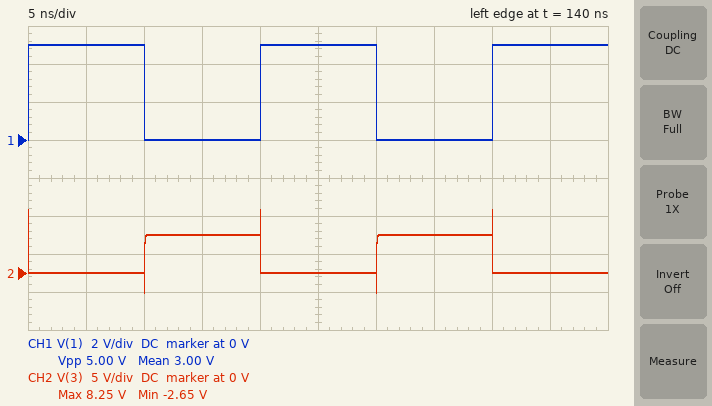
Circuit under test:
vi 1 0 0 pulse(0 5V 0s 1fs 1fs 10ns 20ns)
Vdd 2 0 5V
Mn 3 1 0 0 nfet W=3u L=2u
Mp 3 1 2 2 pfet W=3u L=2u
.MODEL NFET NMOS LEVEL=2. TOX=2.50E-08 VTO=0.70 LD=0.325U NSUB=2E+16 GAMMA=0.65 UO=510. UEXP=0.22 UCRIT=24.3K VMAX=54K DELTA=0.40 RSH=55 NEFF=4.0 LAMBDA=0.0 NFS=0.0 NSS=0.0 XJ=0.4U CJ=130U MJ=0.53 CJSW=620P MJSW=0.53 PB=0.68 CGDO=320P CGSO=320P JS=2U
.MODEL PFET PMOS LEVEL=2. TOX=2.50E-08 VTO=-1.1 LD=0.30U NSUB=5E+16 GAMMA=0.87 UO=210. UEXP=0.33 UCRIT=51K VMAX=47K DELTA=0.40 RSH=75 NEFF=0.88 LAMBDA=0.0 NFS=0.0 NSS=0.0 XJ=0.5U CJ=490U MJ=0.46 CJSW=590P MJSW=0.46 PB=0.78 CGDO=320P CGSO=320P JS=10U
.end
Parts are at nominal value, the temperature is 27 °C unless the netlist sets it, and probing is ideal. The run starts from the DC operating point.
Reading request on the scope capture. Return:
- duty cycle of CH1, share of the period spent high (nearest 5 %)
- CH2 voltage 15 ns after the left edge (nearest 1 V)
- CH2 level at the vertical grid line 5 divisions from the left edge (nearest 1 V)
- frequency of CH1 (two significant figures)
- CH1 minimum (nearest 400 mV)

50 %
5 V
0 V
50 MHz
0 V
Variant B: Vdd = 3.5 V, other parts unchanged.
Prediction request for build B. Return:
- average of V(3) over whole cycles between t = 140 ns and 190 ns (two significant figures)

1.7 V
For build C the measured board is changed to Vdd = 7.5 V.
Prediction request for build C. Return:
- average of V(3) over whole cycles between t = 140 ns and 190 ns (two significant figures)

3.8 V
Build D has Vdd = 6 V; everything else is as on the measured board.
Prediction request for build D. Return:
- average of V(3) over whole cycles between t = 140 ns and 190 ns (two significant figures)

3.0 V
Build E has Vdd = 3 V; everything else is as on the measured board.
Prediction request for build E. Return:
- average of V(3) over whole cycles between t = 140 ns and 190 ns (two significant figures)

1.5 V
